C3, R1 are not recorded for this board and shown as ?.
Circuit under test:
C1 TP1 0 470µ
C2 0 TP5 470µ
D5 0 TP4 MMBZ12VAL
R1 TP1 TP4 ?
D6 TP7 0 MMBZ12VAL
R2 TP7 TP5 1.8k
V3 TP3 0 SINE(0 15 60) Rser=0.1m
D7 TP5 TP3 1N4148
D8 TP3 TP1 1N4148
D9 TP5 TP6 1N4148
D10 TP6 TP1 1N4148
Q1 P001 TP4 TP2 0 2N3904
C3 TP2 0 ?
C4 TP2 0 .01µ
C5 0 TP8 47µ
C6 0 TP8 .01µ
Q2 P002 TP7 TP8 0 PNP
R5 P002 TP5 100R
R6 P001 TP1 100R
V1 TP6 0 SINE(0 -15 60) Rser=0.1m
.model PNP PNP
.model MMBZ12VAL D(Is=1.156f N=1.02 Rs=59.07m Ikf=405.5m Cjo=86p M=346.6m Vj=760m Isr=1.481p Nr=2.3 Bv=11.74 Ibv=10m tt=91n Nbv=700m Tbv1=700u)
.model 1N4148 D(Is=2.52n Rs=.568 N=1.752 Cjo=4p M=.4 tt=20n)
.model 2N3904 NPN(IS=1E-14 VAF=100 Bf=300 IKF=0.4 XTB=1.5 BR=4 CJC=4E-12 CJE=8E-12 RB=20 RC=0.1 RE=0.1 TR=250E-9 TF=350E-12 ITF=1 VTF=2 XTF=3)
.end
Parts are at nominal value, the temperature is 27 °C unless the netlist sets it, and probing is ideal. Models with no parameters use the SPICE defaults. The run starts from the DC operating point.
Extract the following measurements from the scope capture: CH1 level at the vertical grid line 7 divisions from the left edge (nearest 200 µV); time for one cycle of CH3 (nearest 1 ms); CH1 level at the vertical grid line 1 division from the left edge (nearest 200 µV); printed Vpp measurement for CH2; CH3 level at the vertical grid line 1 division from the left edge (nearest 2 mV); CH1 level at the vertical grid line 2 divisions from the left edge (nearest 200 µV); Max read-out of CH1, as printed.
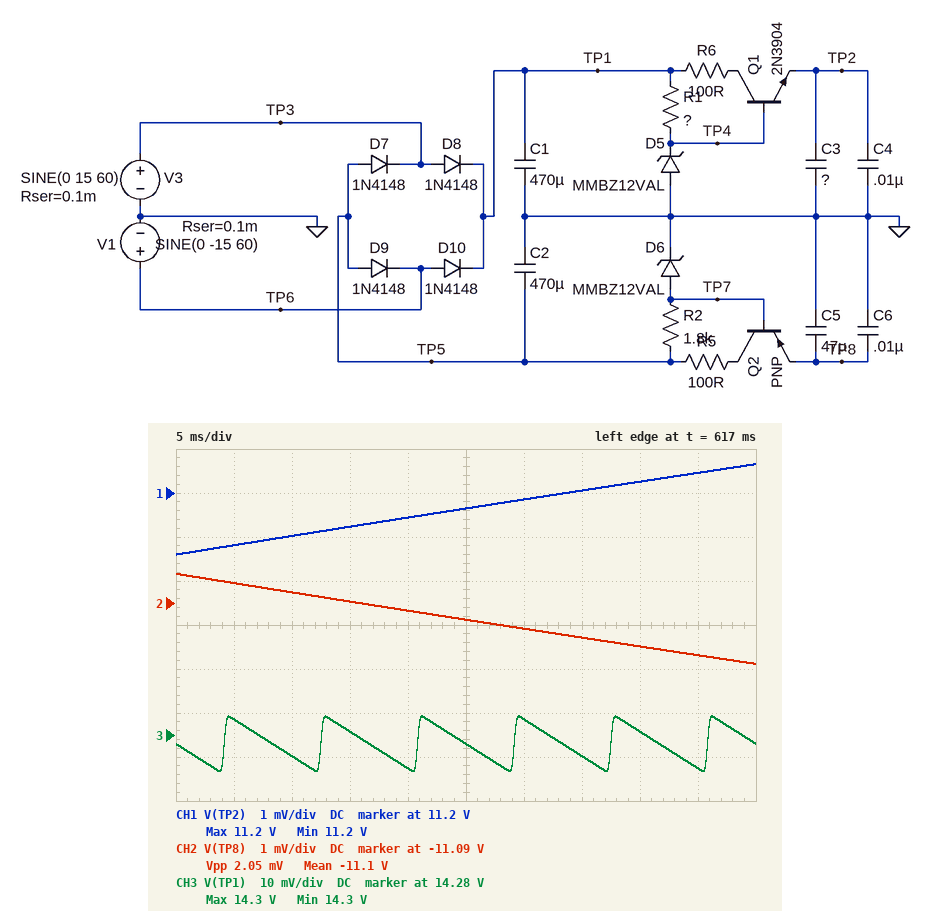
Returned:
11.1970 V
8 ms
11.1958 V
2.05 mV
14.284 V
11.1960 V
11.2 V
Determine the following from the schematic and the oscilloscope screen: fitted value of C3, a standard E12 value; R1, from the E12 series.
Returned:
56 µF
3.3 kΩ
